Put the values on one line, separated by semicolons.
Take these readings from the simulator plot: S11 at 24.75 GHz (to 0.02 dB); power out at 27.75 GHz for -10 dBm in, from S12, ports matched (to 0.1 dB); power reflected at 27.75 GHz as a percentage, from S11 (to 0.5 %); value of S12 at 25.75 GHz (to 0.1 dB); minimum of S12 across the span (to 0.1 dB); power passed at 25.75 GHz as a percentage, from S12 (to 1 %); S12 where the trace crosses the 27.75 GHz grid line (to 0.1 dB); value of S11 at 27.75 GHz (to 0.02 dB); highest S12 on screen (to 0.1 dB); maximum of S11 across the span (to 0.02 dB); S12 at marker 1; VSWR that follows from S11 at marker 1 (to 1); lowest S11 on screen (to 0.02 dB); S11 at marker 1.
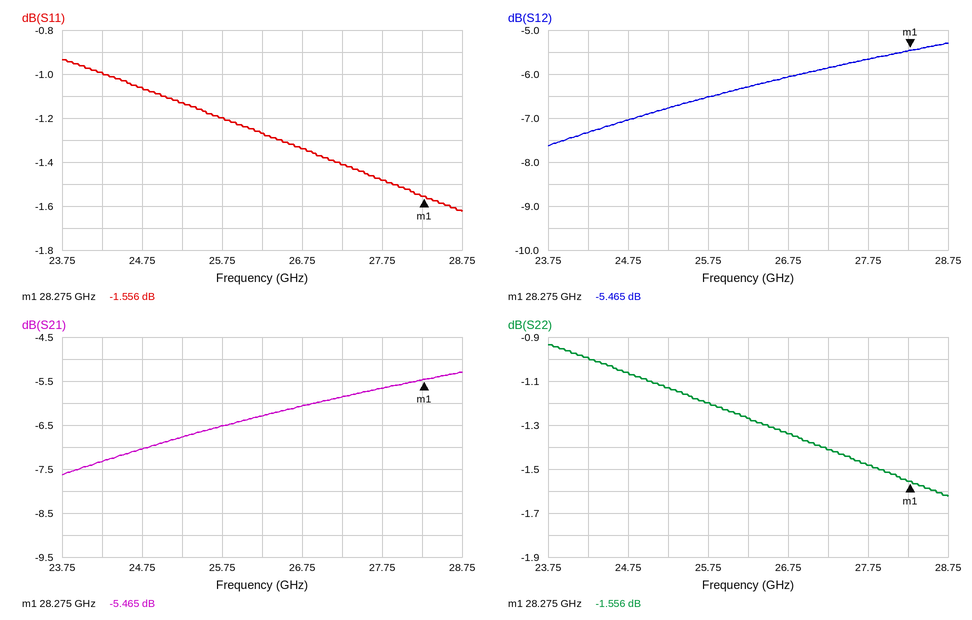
-1.06 dB; -15.7 dBm; 71.0 %; -6.5 dB; -7.6 dB; 22 %; -5.7 dB; -1.48 dB; -5.3 dB; -0.94 dB; -5.465 dB; 11; -1.62 dB; -1.556 dB
